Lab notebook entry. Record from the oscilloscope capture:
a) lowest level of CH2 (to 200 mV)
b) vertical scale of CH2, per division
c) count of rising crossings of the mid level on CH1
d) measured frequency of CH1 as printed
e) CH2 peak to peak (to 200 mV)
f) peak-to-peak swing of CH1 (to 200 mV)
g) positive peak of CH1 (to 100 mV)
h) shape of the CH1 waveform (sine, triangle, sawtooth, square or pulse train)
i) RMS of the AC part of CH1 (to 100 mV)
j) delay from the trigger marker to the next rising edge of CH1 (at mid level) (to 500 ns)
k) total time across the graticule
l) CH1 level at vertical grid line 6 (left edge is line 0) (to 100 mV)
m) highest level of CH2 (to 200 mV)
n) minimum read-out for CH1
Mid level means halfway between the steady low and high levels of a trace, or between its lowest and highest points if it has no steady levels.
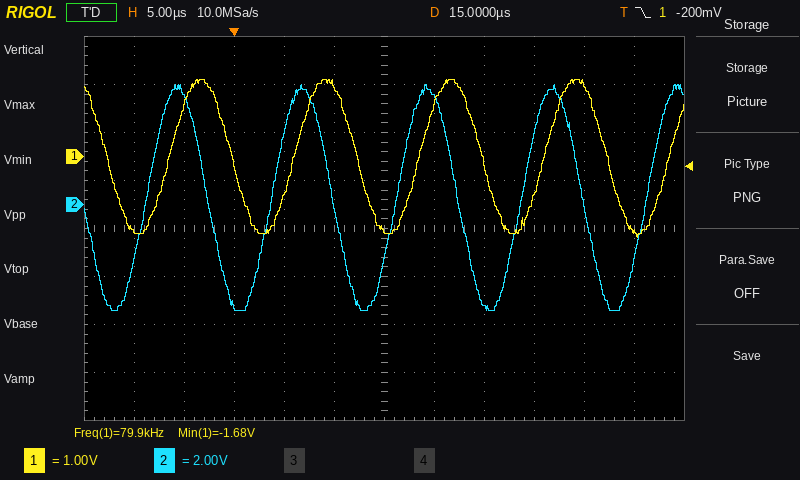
-4.4 V
2 V
5
79.9 kHz
9.4 V
3.2 V
1.6 V
sine
1.1 V
6.0 µs
60 µs
-1.5 V
5.0 V
-1.68 V
